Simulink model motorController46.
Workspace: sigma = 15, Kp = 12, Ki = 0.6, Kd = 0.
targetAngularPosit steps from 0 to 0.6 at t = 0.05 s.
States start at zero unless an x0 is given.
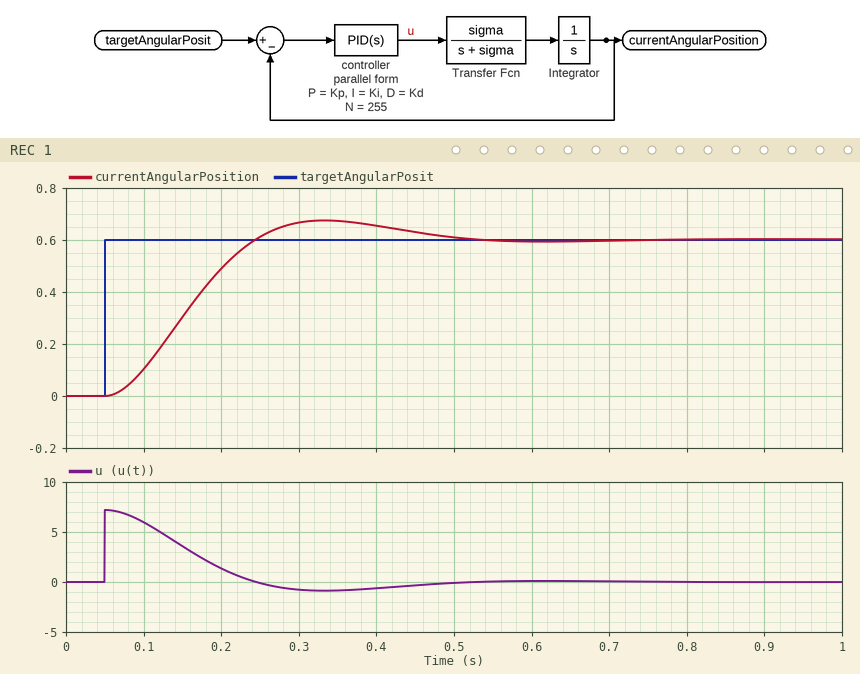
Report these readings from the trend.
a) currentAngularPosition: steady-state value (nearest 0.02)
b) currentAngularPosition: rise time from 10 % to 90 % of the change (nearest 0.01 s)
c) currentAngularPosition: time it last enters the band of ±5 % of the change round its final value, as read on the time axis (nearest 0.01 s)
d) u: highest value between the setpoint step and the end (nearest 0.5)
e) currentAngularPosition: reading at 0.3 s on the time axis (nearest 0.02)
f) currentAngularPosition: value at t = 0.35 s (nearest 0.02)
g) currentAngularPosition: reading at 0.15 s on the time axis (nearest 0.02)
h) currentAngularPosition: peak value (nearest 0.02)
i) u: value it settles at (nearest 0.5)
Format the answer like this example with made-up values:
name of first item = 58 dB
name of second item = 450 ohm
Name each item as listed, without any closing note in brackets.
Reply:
currentAngularPosition: steady-state value = 0.60
currentAngularPosition: rise time from 10 % to 90 % of the change = 0.13 s
currentAngularPosition: time it last enters the band of ±5 % of the change round its final value, as read on the time axis = 0.45 s
u: highest value between the setpoint step and the end = 7.0
currentAngularPosition: reading at 0.3 s on the time axis = 0.66
currentAngularPosition: value at t = 0.35 s = 0.68
currentAngularPosition: reading at 0.15 s on the time axis = 0.30
currentAngularPosition: peak value = 0.68
u: value it settles at = 0.0
